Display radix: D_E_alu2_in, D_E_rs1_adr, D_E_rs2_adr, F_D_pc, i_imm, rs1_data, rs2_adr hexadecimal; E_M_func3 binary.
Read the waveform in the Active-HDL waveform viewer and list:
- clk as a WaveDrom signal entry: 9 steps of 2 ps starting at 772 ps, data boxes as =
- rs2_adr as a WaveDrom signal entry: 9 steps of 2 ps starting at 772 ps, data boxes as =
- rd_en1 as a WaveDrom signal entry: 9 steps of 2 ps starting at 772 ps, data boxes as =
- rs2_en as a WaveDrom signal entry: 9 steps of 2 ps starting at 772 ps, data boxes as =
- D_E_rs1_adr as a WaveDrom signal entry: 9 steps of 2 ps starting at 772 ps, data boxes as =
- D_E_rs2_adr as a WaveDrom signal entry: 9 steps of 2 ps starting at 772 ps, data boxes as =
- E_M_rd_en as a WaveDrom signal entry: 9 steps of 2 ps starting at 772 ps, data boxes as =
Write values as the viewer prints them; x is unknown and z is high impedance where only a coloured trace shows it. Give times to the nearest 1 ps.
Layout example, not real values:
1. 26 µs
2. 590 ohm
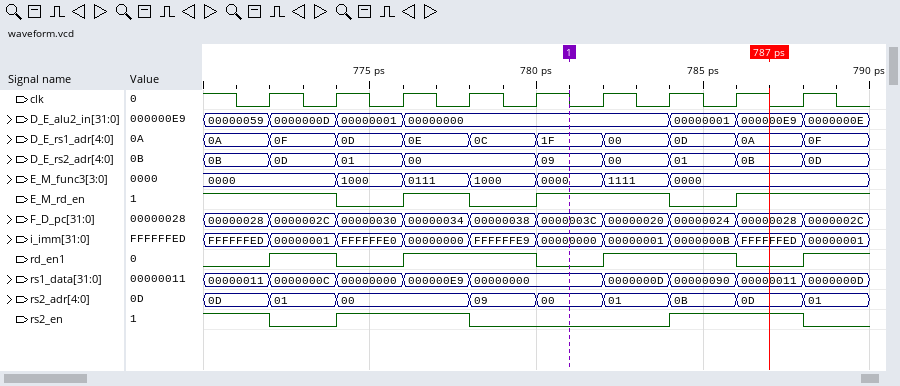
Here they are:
1. {name: 'clk', wave: 'p........'}
2. {name: 'rs2_adr', wave: '==.======', data: '01 00 09 00 01 0B 0D 01'}
3. {name: 'rd_en1', wave: '101.01.01'}
4. {name: 'rs2_en', wave: '01.0..1.0'}
5. {name: 'D_E_rs1_adr', wave: '=========', data: '0F 0D 0E 0C 1F 00 0D 0A 0F'}
6. {name: 'D_E_rs2_adr', wave: '===.=====', data: '0D 01 00 09 00 01 0B 0D'}
7. {name: 'E_M_rd_en', wave: '10101.01.'}
